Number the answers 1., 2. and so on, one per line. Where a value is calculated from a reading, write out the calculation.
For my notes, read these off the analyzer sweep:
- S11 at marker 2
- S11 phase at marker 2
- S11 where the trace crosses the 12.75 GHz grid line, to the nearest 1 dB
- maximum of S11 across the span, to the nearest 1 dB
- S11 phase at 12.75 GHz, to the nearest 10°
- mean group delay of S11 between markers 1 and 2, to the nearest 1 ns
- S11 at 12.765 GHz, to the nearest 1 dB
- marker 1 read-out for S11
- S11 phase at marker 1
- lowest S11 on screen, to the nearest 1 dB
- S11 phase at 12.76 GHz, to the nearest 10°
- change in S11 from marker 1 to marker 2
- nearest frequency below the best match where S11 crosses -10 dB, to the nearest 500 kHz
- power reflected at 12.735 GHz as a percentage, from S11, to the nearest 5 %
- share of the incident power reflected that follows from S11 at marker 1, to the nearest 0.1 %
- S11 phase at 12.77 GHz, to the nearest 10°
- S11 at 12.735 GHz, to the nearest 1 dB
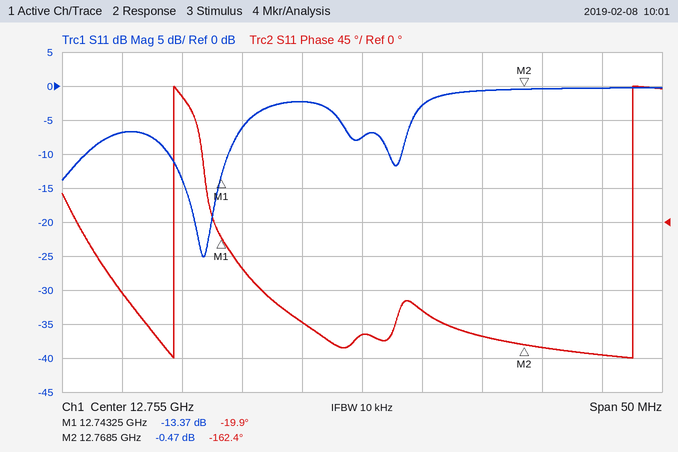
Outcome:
1. -0.47 dB
2. -162.4°
3. -2 dB
4. 0 dB
5. -130°
6. −(-162.4° − (-19.9°))/(360° × 25.25 MHz) ≈ 16 ns
7. -1 dB
8. -13.37 dB
9. -19.9°
10. -25 dB
11. -120°
12. -0.47 − (-13.37) = 12.90 dB
13. 12.7390 GHz
14. 10^(-7/10) ≈ 20 %
15. 10^(-13.37/10) ≈ 4.6 %
16. -170°
17. -7 dB
